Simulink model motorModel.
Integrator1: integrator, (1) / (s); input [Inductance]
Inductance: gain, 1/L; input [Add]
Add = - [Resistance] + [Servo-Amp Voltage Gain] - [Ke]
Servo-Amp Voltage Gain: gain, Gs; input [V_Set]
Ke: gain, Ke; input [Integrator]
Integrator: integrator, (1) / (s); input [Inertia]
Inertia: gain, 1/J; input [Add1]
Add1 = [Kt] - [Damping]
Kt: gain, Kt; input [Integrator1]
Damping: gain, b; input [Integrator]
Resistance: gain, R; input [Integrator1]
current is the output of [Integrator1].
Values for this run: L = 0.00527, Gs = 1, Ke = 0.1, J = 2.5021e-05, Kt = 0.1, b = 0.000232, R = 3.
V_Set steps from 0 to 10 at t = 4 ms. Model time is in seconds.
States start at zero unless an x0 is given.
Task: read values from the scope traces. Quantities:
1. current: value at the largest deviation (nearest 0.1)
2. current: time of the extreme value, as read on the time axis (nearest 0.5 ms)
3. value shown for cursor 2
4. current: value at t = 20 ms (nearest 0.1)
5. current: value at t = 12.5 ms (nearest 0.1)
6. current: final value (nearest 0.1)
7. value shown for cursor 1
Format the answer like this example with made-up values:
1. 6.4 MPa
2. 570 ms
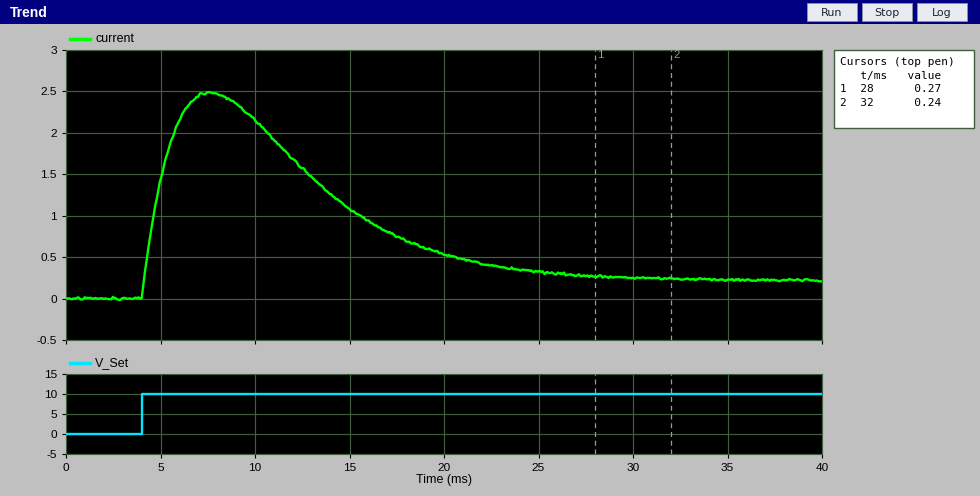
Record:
1. 2.5
2. 7.5 ms
3. 0.24
4. 0.5
5. 1.6
6. 0.2
7. 0.27
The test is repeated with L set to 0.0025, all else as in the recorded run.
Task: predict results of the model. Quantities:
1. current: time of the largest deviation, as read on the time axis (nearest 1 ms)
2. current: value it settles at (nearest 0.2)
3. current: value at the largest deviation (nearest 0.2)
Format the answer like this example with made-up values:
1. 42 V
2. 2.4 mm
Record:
1. 6 ms
2. 0.2
3. 2.8
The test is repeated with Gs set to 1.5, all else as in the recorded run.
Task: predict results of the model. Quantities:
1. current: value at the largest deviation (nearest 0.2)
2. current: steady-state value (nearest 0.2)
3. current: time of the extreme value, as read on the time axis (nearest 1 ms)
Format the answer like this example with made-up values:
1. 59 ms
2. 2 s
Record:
1. 3.8
2. 0.4
3. 8 ms
